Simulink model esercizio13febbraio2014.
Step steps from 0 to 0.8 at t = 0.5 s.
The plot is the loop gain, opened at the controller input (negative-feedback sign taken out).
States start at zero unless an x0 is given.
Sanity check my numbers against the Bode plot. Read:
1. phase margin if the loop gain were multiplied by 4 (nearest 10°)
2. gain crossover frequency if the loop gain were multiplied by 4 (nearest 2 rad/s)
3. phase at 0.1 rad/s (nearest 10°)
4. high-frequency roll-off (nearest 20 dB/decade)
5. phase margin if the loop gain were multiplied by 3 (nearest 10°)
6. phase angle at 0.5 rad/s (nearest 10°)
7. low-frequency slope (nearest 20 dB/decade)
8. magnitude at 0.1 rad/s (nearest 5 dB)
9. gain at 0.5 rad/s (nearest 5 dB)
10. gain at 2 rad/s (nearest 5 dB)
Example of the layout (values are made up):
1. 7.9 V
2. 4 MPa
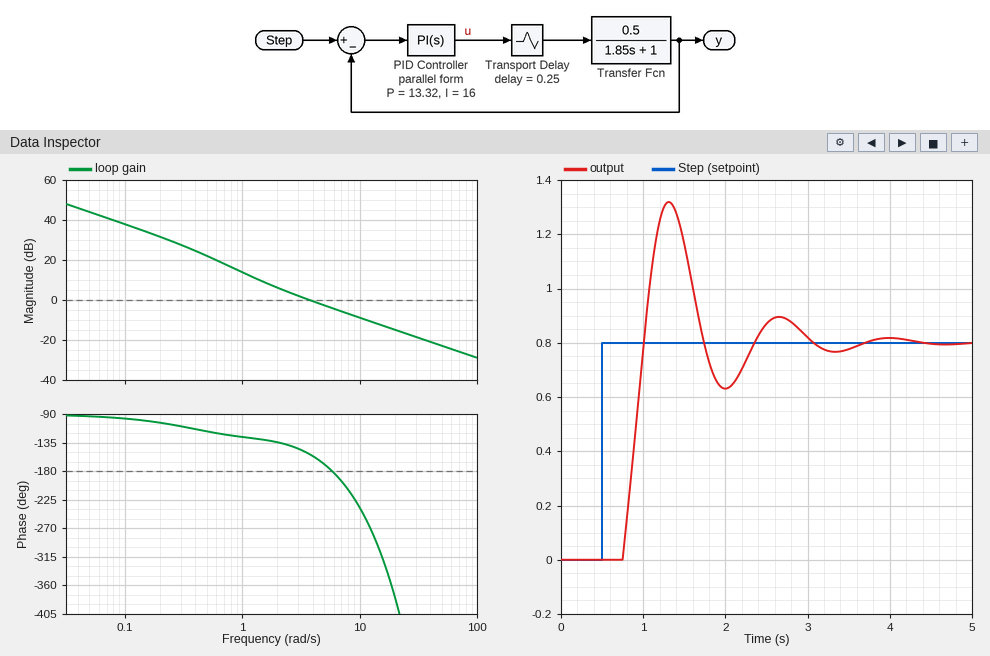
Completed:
1. -120°
2. 14 rad/s
3. -100°
4. -20 dB/decade
5. -70°
6. -120°
7. -20 dB/decade
8. 40 dB
9. 20 dB
10. 5 dB
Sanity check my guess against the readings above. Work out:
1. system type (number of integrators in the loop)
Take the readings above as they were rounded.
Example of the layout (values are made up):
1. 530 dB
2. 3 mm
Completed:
1. 1
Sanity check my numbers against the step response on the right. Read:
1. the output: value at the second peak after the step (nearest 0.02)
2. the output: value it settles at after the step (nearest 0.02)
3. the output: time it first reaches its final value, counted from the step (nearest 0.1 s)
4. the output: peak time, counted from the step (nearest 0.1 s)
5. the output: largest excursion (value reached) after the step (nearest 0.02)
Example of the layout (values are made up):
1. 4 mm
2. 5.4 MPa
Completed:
1. 0.90
2. 0.80
3. 0.5 s
4. 0.8 s
5. 1.32
